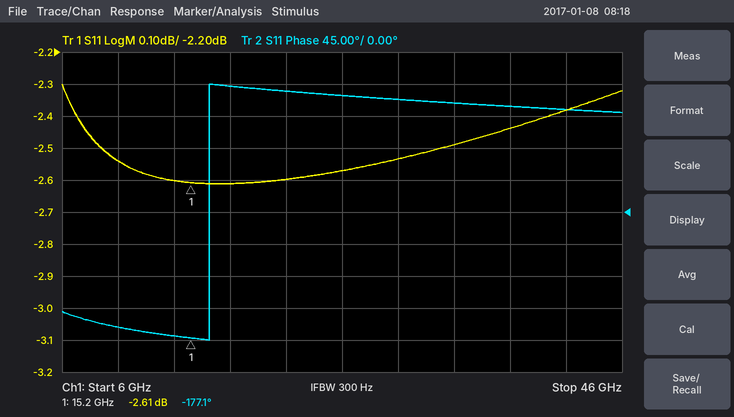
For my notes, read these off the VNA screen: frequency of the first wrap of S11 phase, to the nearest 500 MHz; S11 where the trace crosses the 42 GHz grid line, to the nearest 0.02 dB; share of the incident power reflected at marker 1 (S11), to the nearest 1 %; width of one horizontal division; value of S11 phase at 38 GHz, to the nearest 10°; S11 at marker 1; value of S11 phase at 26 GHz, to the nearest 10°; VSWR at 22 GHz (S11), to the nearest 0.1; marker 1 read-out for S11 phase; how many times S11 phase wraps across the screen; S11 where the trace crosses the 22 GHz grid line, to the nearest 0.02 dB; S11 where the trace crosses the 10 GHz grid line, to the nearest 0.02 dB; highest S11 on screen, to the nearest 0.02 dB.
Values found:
16.5 GHz
-2.38 dB
55 %
4 GHz
150°
-2.61 dB
160°
6.7
-177.1°
1
-2.60 dB
-2.54 dB
-2.30 dB
